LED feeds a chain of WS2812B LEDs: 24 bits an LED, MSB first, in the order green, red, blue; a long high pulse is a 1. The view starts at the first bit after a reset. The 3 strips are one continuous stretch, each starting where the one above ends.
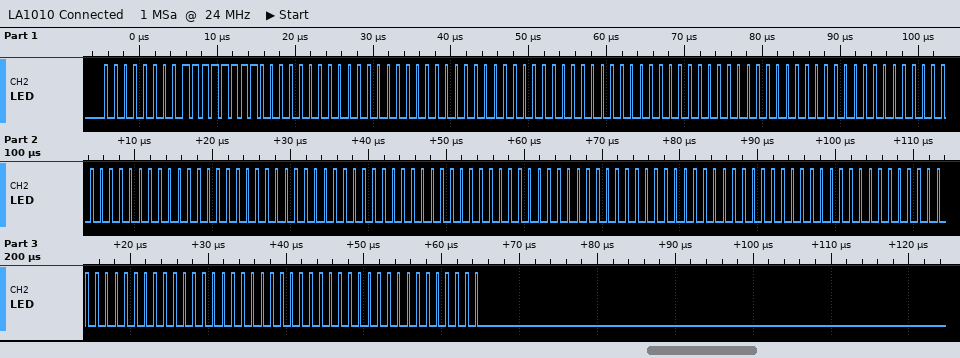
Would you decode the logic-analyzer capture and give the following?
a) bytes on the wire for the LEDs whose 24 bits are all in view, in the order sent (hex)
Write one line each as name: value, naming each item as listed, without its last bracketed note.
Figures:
bytes on the wire for the LEDs whose 24 bits are all in view, in the order sent: 00 FF 00 00 00 00 00 00 00 00 00 00 00 00 00 00 00 00 00 00 00 00 00 00 00 00 00
